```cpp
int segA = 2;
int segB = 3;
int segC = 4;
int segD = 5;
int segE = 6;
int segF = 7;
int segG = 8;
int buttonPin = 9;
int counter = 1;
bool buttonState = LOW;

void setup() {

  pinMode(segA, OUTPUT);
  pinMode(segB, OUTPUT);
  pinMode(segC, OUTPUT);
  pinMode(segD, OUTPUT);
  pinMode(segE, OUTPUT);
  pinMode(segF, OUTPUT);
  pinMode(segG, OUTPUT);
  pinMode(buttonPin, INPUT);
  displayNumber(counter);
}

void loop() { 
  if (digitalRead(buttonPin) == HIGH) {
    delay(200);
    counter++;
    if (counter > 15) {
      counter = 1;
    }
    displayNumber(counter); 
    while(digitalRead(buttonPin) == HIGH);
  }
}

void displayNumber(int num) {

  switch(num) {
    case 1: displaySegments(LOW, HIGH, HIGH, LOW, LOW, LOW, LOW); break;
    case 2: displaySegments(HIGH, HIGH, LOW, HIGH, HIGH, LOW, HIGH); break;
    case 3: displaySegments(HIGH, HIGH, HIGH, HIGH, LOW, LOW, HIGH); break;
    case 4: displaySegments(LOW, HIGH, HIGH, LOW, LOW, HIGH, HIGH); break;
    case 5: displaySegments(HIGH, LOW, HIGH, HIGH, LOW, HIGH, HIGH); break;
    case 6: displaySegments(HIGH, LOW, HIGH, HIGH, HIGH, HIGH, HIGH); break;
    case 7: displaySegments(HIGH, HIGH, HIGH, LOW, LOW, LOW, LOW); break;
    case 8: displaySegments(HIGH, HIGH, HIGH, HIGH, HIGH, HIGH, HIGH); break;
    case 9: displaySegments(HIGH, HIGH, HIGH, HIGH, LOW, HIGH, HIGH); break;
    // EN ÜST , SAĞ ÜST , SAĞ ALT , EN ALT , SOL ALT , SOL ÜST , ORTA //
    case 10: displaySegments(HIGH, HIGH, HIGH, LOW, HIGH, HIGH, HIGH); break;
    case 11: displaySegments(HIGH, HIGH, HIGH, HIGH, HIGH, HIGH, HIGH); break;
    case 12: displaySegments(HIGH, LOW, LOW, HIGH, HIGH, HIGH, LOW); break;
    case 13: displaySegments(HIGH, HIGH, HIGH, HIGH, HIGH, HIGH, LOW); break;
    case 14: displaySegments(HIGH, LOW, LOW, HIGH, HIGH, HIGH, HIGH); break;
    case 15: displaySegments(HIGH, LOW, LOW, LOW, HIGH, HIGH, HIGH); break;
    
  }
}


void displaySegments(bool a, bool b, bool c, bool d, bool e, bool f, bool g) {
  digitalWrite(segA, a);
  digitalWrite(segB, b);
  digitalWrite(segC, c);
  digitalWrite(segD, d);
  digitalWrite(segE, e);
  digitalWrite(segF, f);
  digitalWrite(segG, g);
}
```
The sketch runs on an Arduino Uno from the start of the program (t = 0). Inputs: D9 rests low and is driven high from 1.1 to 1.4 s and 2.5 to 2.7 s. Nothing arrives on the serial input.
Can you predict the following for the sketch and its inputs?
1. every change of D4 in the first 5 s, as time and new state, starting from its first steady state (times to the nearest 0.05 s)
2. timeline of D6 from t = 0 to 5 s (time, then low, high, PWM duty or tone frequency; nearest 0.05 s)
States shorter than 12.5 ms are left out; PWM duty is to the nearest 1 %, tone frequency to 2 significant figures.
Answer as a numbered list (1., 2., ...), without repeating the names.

1. 0 s high; 1.3 s low; 2.7 s high
2. 0 s low; 1.3 s high; 2.7 s low
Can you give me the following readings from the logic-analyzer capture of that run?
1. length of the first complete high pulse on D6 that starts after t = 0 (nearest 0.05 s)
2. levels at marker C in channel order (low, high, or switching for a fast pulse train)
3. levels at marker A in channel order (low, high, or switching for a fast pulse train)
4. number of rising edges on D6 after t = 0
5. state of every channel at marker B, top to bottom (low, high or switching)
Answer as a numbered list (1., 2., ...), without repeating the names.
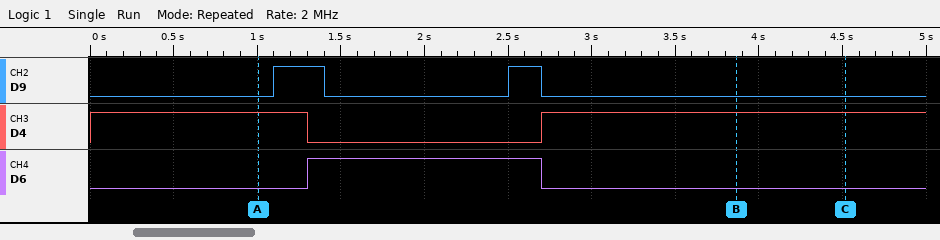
1. 1.40 s
2. D9 low, D4 high, D6 low
3. D9 low, D4 high, D6 low
4. 1
5. D9 low, D4 high, D6 low
